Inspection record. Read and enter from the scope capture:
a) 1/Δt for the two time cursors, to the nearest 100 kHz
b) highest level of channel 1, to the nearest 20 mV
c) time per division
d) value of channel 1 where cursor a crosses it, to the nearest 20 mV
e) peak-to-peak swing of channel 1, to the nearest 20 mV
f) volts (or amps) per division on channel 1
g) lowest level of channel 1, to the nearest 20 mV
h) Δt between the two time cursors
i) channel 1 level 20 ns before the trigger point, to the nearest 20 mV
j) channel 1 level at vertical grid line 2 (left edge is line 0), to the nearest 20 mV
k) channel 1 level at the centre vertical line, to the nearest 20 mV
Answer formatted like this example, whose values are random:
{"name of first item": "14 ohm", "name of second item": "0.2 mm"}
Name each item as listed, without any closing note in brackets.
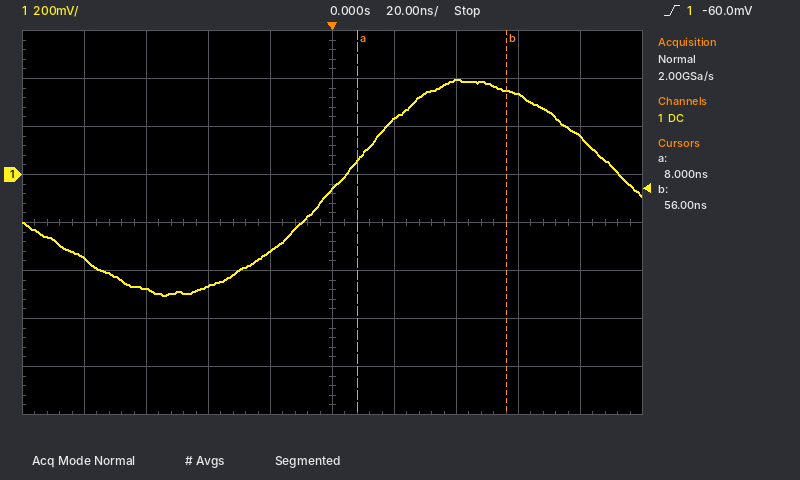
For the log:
{"1/Δt for the two time cursors, to the nearest 100 kHz": "20.8 MHz", "highest level of channel 1, to the nearest 20 mV": "400 mV", "time per division": "20 ns", "value of channel 1 where cursor a crosses it, to the nearest 20 mV": "60 mV", "peak-to-peak swing of channel 1, to the nearest 20 mV": "900 mV", "volts (or amps) per division on channel 1": "200 mV", "lowest level of channel 1, to the nearest 20 mV": "-500 mV", "Δt between the two time cursors": "48 ns", "channel 1 level 20 ns before the trigger point, to the nearest 20 mV": "-320 mV", "channel 1 level at vertical grid line 2 (left edge is line 0), to the nearest 20 mV": "-480 mV", "channel 1 level at the centre vertical line, to the nearest 20 mV": "-60 mV"}
